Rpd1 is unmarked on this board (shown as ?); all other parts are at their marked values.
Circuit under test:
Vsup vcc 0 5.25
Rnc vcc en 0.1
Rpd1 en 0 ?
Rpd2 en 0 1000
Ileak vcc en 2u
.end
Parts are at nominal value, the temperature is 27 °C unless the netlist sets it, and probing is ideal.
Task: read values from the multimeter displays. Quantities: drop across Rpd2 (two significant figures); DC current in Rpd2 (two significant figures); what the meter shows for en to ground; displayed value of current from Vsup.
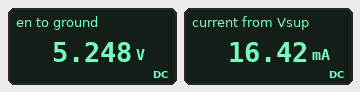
5.2 V
5.2 mA
5.248 V
16.42 mA
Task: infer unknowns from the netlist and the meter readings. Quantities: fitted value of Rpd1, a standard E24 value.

470 Ω
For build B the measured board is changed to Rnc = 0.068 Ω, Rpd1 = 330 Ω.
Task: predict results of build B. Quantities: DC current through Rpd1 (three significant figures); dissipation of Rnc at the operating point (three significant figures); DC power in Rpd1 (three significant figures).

15.9 mA
30.4 µW
83.5 mW
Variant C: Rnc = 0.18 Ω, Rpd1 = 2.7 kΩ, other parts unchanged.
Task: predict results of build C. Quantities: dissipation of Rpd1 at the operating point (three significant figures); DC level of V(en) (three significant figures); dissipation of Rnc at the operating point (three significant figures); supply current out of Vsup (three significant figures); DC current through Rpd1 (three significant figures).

10.2 mW
5.25 V
9.31 µW
7.19 mA
1.94 mA
